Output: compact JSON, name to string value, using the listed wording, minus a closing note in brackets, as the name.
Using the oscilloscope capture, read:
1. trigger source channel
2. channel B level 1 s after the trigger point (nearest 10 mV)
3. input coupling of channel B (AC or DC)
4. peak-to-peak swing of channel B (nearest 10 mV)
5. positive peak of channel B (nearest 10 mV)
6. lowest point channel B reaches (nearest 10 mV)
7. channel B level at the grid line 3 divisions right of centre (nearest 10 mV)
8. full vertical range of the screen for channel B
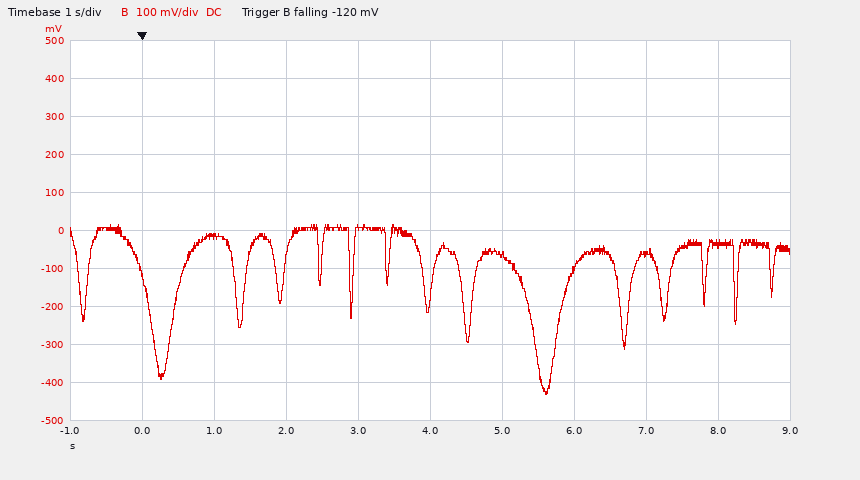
{"trigger source channel": "channel B", "channel B level 1 s after the trigger point": "-20 mV", "input coupling of channel B": "DC", "peak-to-peak swing of channel B": "450 mV", "positive peak of channel B": "20 mV", "lowest point channel B reaches": "-430 mV", "channel B level at the grid line 3 divisions right of centre": "-60 mV", "full vertical range of the screen for channel B": "1 V"}
